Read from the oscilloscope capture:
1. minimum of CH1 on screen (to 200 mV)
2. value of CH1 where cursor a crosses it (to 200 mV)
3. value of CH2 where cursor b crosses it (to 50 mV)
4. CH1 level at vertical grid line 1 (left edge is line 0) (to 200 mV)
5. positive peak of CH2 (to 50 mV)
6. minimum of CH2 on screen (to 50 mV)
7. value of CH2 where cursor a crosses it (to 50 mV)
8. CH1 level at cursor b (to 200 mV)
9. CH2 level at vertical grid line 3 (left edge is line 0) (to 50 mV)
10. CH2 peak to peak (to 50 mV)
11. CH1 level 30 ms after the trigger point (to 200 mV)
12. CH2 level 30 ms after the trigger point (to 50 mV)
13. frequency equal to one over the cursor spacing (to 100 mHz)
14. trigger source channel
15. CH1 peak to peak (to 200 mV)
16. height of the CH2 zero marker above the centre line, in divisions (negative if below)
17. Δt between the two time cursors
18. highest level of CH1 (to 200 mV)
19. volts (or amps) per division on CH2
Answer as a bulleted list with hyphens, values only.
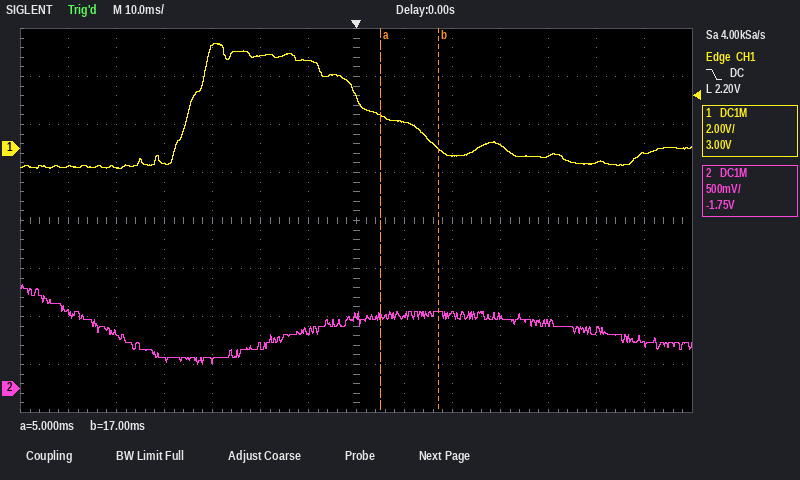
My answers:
- -800 mV
- 1.4 V
- 800 mV
- -800 mV
- 1.10 V
- 250 mV
- 750 mV
- 0.0 V
- 300 mV
- 850 mV
- 200 mV
- 750 mV
- 83.3 Hz
- CH1
- 5.2 V
- -3.5 div
- 12 ms
- 4.4 V
- 500 mV
